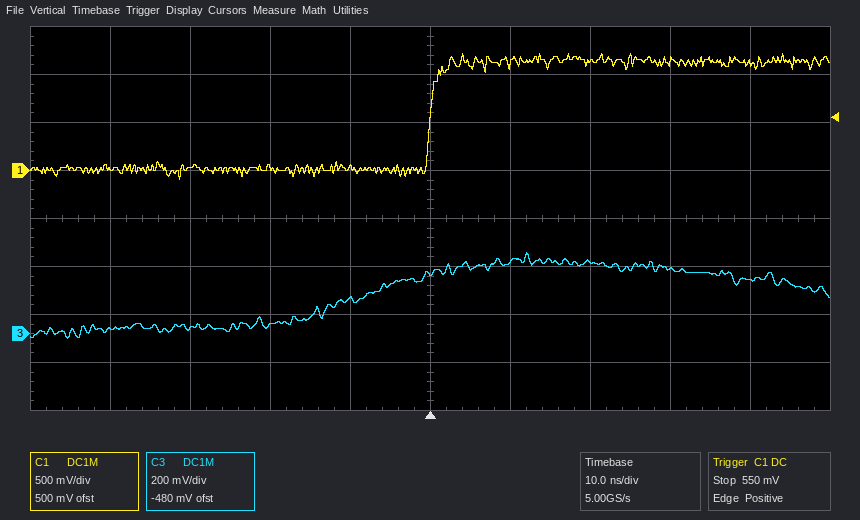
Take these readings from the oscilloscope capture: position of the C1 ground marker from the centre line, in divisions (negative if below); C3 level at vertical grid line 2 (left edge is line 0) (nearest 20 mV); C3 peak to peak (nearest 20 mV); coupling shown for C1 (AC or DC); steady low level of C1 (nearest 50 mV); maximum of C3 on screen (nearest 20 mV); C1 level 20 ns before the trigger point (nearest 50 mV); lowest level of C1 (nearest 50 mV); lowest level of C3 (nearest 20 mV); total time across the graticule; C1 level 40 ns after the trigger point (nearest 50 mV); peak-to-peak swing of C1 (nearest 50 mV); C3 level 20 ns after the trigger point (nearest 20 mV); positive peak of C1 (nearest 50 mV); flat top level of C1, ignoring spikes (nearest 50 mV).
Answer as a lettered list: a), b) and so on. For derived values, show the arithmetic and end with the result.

a) +1.0 div
b) 20 mV
c) 340 mV − (-20 mV) = 360 mV
d) DC
e) 0 mV
f) 340 mV
g) 50 mV
h) -100 mV
i) -20 mV
j) 100 ns
k) 1.10 V
l) 1.20 V − (-100 mV) = 1.30 V
m) 300 mV
n) 1.20 V
o) 1.15 V
